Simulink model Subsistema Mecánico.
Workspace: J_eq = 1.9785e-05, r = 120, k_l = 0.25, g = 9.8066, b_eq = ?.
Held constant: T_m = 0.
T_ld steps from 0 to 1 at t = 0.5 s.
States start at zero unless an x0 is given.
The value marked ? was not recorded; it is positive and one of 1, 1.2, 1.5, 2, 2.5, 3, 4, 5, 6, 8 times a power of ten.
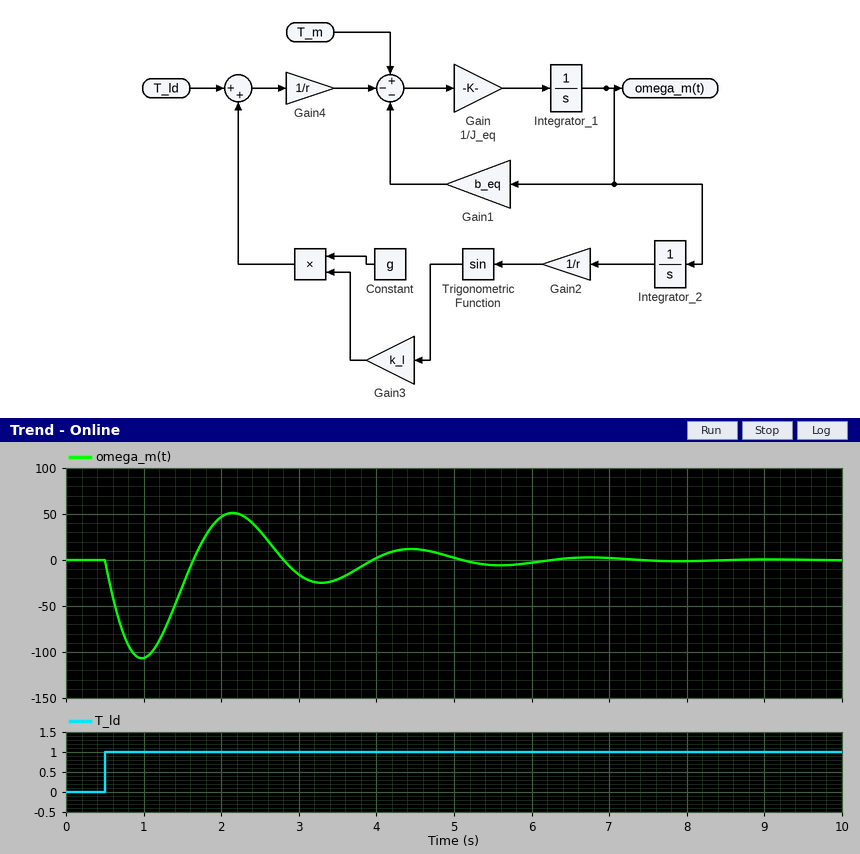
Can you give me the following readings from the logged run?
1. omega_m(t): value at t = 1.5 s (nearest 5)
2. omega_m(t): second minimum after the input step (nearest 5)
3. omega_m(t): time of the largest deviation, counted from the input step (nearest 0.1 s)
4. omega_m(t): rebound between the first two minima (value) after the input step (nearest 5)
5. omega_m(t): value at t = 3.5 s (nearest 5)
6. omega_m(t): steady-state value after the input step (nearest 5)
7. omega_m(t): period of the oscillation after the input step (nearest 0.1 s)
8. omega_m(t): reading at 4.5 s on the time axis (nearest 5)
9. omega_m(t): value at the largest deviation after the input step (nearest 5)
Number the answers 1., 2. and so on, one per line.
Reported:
1. -30
2. -25
3. 0.5 s
4. 50
5. -20
6. 0
7. 2.3 s
8. 10
9. -105
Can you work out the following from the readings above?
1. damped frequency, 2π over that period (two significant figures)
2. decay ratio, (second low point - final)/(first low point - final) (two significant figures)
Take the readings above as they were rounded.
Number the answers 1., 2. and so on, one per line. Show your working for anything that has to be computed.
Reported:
1. 2π / 2.3 = 2.7 rad/s
2. (-25 - 0) / (-105 - 0) = 0.24
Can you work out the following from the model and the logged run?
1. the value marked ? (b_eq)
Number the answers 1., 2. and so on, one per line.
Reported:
1. 2.5e-05
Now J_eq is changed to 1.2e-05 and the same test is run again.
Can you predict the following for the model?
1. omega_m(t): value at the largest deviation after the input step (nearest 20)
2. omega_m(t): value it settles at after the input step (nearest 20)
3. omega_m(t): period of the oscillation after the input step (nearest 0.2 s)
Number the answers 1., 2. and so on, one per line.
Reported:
1. -120
2. 0
3. 1.8 s
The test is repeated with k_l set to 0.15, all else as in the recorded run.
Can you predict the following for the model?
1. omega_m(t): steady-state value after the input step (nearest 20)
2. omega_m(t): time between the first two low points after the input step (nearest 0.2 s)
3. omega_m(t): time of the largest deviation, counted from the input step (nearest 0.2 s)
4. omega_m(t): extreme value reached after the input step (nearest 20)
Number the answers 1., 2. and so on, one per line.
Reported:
1. 0
2. 3.4 s
3. 0.6 s
4. -120
